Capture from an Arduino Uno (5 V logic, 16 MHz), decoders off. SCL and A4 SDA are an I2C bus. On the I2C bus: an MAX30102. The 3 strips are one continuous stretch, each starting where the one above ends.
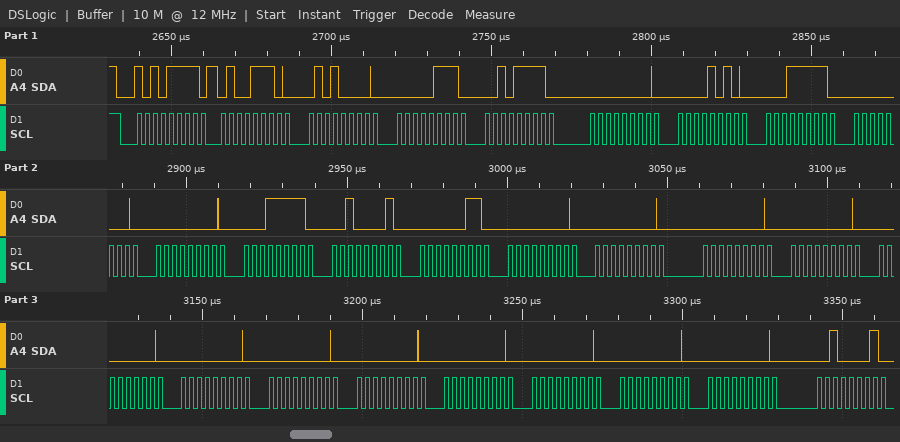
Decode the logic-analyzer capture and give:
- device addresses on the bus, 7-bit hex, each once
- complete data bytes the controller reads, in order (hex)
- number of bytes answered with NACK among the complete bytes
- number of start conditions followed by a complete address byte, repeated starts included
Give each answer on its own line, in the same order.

0x57
4E 50 07 2F 00 0A 1F 00 00 1F 21 03 00 00 00 00 00 00 00 00 00 00 00 00 21
0
1
